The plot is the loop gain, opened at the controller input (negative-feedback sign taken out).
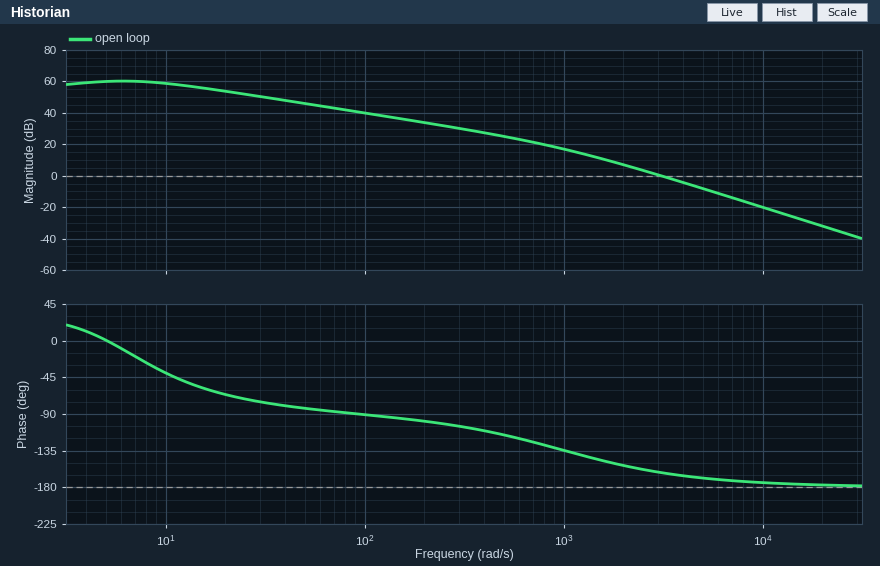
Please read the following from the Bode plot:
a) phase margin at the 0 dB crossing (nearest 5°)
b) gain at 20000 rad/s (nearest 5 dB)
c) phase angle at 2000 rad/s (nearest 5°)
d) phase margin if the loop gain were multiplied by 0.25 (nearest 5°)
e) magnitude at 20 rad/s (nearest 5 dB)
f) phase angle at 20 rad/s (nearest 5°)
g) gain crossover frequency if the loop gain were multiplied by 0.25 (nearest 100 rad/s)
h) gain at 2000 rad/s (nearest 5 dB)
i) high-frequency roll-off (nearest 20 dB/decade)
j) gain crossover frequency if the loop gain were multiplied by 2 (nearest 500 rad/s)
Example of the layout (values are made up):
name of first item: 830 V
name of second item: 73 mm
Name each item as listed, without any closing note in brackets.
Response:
phase margin at the 0 dB crossing: 20°
gain at 20000 rad/s: -30 dB
phase angle at 2000 rad/s: -155°
phase margin if the loop gain were multiplied by 0.25: 35°
magnitude at 20 rad/s: 55 dB
phase angle at 20 rad/s: -65°
gain crossover frequency if the loop gain were multiplied by 0.25: 1400 rad/s
gain at 2000 rad/s: 5 dB
high-frequency roll-off: -40 dB/decade
gain crossover frequency if the loop gain were multiplied by 2: 4500 rad/s
